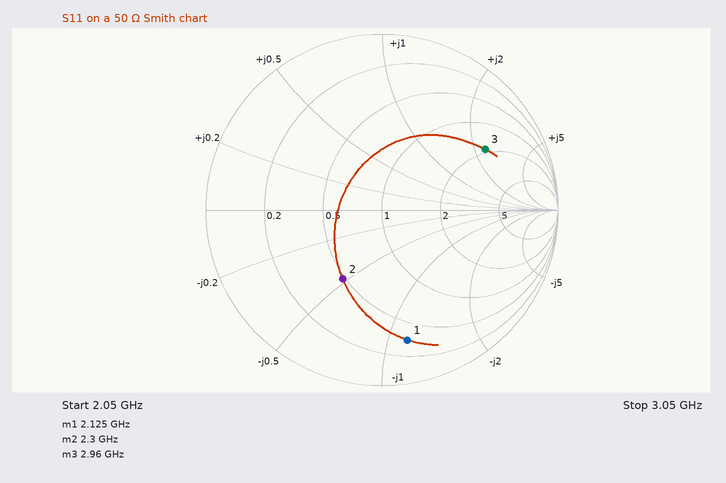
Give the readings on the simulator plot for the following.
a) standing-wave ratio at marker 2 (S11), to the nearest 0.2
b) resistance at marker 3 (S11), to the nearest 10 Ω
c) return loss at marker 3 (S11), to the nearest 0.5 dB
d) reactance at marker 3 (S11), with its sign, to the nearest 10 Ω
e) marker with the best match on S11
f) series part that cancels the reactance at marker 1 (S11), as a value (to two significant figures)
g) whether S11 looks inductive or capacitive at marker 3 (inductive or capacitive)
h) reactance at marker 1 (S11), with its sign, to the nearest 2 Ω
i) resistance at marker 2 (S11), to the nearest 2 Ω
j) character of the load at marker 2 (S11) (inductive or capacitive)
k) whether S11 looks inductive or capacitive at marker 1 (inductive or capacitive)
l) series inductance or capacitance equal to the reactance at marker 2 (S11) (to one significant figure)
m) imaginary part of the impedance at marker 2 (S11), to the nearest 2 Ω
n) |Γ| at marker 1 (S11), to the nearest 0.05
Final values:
2.6
90 Ω
3.5 dB
+120 Ω
marker 2
4.3 nH
inductive
-58 Ω
24 Ω
capacitive
capacitive
3 pF
-24 Ω
0.75
